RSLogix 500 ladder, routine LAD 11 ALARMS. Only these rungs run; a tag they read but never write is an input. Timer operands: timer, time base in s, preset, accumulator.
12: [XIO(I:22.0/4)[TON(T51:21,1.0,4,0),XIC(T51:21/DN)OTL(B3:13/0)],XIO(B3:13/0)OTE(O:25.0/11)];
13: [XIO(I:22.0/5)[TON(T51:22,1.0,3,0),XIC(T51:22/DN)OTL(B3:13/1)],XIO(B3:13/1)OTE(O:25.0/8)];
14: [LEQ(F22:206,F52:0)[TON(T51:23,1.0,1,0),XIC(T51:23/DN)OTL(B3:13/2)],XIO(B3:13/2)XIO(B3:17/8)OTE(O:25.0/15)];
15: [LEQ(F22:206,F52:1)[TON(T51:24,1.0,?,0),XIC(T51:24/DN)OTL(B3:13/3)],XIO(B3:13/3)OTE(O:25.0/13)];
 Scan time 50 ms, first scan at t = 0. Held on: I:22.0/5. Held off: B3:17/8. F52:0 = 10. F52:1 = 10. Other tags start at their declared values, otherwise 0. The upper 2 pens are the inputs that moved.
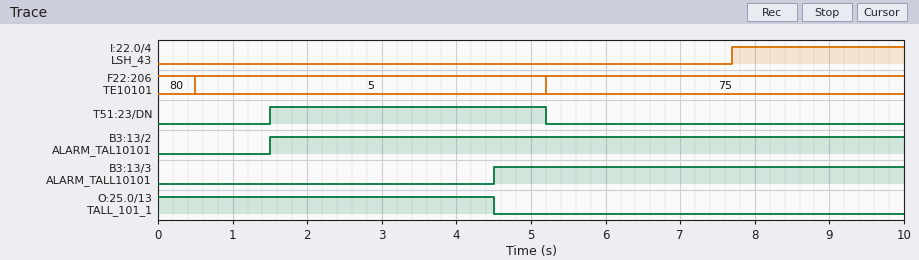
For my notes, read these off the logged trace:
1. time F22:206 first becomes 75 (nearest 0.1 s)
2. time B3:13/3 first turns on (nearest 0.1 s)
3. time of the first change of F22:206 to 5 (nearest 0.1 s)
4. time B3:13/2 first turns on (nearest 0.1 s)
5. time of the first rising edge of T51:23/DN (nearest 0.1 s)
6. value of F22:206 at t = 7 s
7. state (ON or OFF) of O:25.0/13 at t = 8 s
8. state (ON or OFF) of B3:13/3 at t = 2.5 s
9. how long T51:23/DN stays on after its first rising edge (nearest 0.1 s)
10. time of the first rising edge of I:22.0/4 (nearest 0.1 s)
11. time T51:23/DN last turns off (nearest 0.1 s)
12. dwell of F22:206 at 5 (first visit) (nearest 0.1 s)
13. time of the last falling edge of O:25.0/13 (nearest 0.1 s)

5.2 s
4.5 s
0.5 s
1.5 s
1.5 s
75
OFF
OFF
3.7 s
7.7 s
5.2 s
4.7 s
4.5 s
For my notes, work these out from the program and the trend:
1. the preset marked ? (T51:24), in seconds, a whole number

4 s
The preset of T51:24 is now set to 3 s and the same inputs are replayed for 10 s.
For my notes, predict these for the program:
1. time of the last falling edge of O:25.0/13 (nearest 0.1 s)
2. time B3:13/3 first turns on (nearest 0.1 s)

3.5 s
3.5 s
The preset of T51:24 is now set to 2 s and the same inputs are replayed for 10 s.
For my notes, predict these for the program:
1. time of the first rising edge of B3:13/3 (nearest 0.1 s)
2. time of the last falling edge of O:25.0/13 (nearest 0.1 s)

2.5 s
2.5 s
